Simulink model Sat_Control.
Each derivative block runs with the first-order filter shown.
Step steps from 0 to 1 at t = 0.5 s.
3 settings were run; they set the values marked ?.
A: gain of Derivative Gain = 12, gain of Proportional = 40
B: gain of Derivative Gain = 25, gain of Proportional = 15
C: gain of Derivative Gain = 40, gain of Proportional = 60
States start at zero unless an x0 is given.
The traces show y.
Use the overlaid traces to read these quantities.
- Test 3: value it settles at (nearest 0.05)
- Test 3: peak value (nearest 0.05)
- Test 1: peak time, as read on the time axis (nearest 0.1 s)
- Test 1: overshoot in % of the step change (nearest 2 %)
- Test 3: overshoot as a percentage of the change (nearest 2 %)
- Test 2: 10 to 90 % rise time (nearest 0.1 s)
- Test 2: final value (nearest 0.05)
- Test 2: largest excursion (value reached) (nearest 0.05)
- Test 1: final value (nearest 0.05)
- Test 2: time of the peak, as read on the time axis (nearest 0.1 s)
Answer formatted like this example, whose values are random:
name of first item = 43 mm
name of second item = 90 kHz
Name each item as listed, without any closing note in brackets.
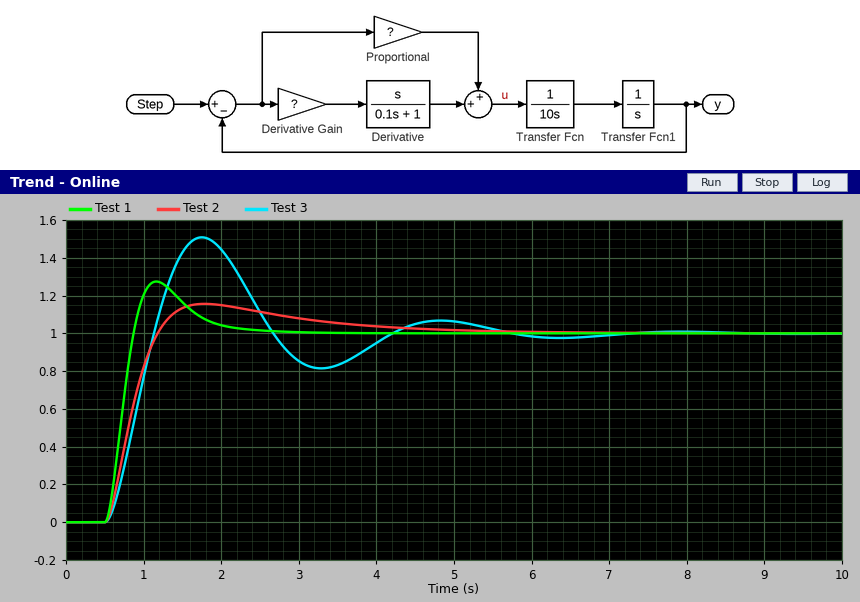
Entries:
Test 3: value it settles at = 1.00
Test 3: peak value = 1.50
Test 1: peak time, as read on the time axis = 1.2 s
Test 1: overshoot in % of the step change = 28 %
Test 3: overshoot as a percentage of the change = 50 %
Test 2: 10 to 90 % rise time = 0.5 s
Test 2: final value = 1.00
Test 2: largest excursion (value reached) = 1.15
Test 1: final value = 1.00
Test 2: time of the peak, as read on the time axis = 1.8 s
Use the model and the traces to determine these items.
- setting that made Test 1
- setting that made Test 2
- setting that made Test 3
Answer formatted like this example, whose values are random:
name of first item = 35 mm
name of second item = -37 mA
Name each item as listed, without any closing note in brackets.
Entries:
setting that made Test 1 = C
setting that made Test 2 = B
setting that made Test 3 = A
